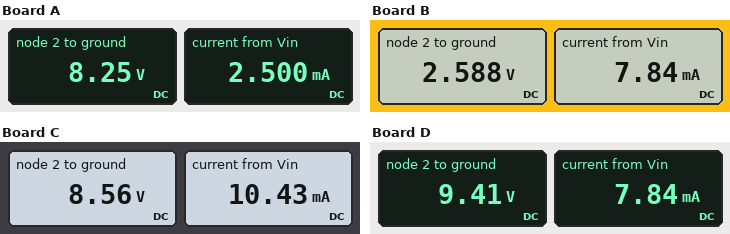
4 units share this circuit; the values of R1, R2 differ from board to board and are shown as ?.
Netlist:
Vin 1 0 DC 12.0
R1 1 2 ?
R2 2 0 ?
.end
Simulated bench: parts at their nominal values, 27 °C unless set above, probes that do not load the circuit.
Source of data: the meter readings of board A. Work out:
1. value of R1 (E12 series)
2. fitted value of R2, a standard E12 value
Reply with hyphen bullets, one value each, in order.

- 1.5 kΩ
- 3.3 kΩ
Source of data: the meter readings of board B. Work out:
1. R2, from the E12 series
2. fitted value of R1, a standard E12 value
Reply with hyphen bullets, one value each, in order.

- 330 Ω
- 1.2 kΩ
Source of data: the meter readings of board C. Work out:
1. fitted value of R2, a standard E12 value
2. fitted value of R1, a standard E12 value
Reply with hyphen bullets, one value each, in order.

- 820 Ω
- 330 Ω
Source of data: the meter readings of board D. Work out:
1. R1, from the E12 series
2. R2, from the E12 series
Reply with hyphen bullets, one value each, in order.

- 330 Ω
- 1.2 kΩ
